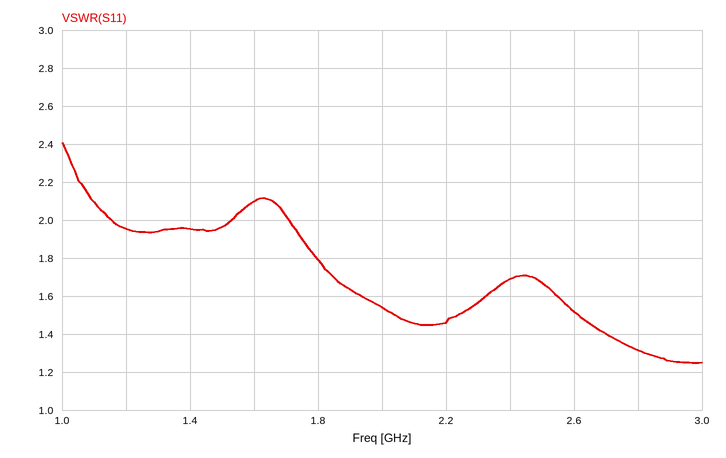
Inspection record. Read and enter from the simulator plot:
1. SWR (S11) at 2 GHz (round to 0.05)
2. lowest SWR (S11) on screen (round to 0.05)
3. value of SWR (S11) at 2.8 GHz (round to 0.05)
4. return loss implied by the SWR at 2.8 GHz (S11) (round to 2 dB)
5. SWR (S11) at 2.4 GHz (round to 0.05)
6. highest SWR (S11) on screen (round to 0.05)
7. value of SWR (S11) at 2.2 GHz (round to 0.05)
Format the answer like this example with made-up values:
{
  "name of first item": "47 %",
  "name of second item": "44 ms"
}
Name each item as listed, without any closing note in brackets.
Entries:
{
  "SWR (S11) at 2 GHz": "1.55",
  "lowest SWR (S11) on screen": "1.25",
  "value of SWR (S11) at 2.8 GHz": "1.30",
  "return loss implied by the SWR at 2.8 GHz (S11)": "18 dB",
  "SWR (S11) at 2.4 GHz": "1.70",
  "highest SWR (S11) on screen": "2.40",
  "value of SWR (S11) at 2.2 GHz": "1.45"
}
